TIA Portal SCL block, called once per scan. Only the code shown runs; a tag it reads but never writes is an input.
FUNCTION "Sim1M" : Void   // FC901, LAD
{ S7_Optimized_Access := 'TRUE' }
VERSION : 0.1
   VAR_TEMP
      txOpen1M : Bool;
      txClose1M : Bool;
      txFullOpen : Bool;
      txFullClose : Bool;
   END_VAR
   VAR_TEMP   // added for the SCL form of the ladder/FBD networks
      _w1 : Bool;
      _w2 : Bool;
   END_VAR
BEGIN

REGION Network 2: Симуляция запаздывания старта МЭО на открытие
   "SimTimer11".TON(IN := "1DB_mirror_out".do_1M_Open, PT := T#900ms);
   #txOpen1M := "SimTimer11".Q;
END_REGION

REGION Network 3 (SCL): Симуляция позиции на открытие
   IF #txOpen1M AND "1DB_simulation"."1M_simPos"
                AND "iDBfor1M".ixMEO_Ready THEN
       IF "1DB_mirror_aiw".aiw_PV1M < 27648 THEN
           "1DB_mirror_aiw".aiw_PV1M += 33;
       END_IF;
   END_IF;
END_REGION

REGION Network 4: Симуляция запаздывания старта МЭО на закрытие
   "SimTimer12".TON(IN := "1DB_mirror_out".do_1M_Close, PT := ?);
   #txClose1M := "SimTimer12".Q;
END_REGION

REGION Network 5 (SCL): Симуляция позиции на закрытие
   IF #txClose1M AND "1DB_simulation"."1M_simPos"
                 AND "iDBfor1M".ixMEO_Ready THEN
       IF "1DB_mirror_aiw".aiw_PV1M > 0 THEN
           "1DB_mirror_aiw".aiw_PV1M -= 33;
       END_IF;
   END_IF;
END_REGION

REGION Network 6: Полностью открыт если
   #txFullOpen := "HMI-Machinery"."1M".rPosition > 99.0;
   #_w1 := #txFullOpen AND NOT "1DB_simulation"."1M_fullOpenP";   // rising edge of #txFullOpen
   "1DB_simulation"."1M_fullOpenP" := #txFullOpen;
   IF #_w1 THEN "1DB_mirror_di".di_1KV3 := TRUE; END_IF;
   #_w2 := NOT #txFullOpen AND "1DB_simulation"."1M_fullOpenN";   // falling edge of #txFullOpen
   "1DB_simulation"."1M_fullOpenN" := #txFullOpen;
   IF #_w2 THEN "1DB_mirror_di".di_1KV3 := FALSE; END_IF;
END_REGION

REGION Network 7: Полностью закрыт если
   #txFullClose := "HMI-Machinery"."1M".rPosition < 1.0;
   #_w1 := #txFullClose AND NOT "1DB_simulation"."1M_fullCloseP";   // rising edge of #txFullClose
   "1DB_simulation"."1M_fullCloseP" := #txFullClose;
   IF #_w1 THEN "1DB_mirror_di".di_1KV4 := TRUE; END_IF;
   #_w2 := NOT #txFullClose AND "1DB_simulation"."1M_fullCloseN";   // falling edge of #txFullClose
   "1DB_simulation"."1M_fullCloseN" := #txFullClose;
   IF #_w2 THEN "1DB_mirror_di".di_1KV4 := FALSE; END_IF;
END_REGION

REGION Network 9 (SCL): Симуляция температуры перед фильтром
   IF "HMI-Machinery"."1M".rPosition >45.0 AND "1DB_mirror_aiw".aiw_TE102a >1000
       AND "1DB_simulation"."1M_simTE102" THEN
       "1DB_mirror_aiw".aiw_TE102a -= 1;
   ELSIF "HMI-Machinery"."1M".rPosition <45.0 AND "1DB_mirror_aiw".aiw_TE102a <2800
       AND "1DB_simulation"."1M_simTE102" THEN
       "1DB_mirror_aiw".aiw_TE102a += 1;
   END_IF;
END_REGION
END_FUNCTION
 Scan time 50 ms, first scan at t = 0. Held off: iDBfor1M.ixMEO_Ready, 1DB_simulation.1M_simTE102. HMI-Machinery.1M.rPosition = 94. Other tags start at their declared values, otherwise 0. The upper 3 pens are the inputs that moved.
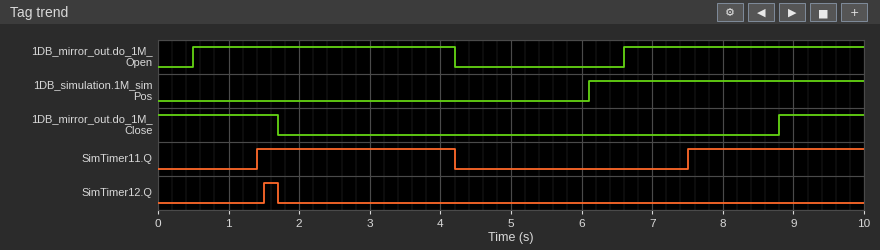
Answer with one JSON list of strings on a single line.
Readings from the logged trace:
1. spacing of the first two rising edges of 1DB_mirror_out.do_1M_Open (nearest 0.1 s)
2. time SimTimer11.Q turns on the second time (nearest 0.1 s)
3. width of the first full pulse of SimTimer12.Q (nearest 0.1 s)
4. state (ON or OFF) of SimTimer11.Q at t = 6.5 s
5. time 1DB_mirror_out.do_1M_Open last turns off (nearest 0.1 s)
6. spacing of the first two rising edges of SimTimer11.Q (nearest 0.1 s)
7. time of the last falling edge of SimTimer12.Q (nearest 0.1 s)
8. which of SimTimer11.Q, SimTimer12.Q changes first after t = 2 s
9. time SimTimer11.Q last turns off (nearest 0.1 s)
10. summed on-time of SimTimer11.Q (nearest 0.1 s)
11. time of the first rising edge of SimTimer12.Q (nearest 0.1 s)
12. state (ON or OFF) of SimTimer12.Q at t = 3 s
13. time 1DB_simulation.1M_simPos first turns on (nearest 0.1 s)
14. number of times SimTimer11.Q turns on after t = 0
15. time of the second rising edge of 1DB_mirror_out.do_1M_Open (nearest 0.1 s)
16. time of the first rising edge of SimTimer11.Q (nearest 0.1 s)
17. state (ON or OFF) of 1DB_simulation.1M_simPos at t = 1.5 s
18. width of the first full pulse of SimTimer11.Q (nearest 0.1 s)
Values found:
["6.1 s", "7.5 s", "0.2 s", "OFF", "4.2 s", "6.1 s", "1.7 s", "SimTimer11.Q", "4.2 s", "5.3 s", "1.5 s", "OFF", "6.1 s", "2", "6.6 s", "1.4 s", "OFF", "2.8 s"]
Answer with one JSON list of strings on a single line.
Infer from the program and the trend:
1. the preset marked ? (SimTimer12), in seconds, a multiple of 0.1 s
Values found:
["1.5 s"]
